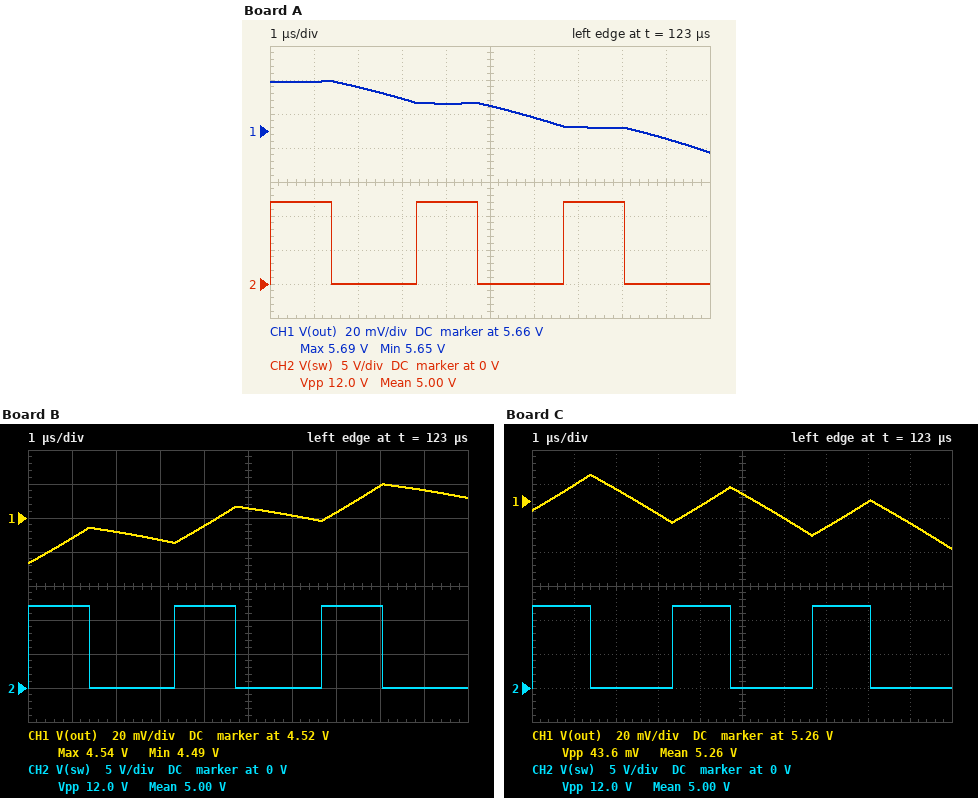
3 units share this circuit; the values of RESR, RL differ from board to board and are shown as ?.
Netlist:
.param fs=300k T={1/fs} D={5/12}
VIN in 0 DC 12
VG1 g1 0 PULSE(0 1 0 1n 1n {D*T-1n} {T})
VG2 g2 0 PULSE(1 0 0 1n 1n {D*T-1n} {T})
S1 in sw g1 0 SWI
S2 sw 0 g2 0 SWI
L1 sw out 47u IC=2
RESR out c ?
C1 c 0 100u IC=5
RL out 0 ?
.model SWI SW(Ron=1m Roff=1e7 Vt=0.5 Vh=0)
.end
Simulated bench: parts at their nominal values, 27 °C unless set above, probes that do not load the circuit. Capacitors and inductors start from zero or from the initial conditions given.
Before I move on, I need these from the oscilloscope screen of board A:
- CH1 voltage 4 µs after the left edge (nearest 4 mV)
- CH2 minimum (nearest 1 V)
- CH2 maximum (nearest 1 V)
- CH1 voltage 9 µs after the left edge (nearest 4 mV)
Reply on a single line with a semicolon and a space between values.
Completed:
5.676 V; 0 V; 12 V; 5.656 V
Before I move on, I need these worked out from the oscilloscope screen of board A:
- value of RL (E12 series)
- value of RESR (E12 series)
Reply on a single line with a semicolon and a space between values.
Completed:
5.6 Ω; 0.027 Ω
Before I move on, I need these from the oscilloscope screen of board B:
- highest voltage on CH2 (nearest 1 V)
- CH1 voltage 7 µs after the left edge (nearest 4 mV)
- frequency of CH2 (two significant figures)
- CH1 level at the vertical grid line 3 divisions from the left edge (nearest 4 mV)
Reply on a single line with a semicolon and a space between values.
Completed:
12 V; 4.524 V; 300 kHz; 4.508 V
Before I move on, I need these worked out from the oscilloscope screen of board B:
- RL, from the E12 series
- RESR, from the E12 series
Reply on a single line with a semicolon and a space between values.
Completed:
1.5 Ω; 0.082 Ω
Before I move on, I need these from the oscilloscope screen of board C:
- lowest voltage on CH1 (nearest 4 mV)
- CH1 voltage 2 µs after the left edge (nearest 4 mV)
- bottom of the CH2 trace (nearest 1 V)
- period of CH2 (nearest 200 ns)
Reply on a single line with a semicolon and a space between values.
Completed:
5.232 V; 5.268 V; 0 V; 3.4 µs
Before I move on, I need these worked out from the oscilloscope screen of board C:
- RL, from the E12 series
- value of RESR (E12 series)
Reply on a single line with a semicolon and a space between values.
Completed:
3.3 Ω; 0.12 Ω
